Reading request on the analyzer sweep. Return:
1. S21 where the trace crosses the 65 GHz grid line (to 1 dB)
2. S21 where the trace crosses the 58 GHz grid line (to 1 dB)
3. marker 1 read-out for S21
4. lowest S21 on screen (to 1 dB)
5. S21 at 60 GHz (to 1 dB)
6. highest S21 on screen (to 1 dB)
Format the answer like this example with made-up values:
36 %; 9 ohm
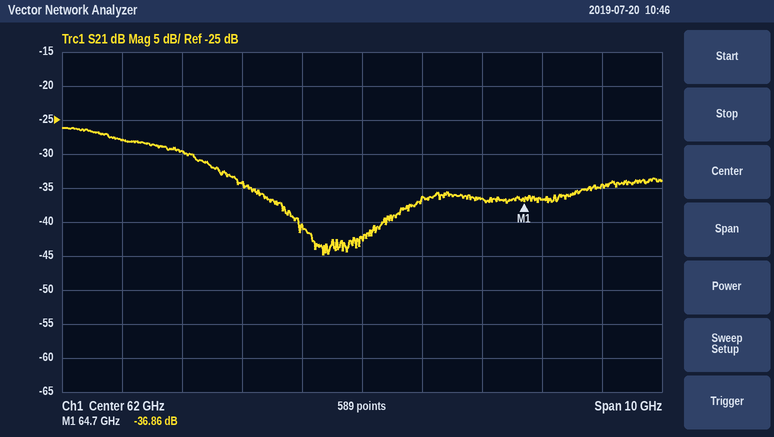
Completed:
-37 dB; -28 dB; -36.86 dB; -45 dB; -34 dB; -26 dB
